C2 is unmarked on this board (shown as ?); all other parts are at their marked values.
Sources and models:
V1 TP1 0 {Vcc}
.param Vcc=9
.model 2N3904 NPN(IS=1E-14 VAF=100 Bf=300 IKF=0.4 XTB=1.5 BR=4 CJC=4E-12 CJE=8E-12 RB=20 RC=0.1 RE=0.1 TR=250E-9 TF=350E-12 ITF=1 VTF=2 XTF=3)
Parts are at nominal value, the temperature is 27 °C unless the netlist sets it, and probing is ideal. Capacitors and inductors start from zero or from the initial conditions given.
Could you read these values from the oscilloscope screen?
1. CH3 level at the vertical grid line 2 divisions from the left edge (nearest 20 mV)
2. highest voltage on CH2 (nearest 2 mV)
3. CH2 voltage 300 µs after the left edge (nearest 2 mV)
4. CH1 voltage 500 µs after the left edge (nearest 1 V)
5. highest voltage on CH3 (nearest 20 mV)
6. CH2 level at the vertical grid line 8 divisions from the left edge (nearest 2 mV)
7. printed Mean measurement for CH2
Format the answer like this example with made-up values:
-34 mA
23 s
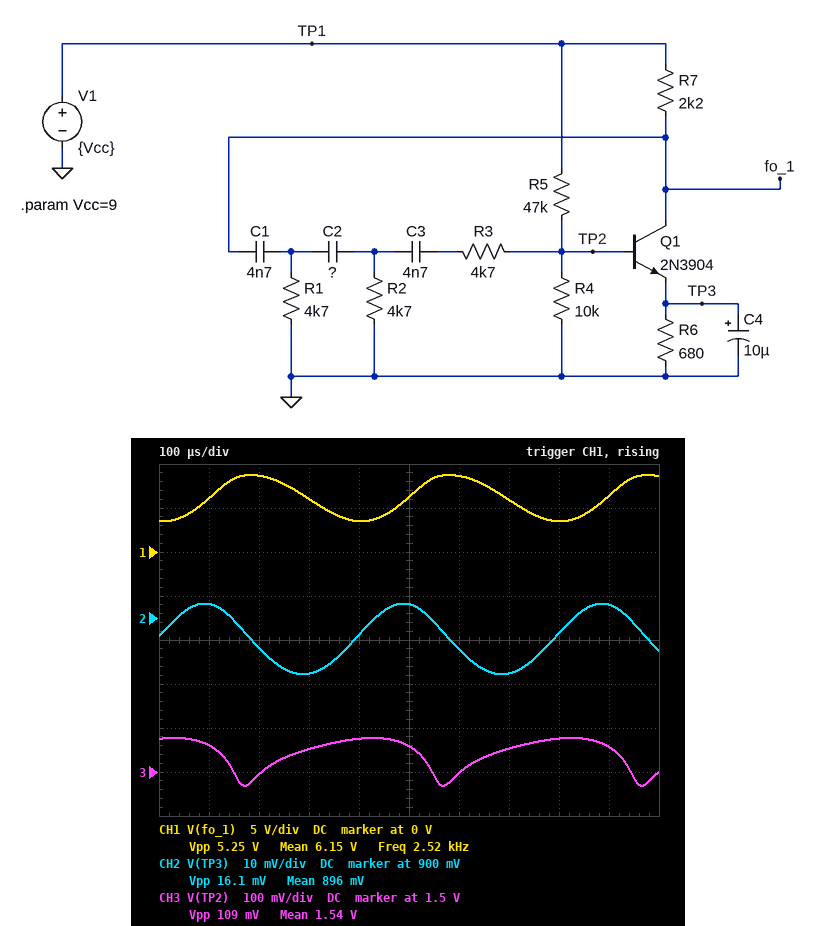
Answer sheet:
1.50 V
904 mV
888 mV
6 V
1.58 V
896 mV
896 mV
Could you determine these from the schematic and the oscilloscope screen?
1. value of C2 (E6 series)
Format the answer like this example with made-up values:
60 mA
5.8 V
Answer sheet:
3.3 nF
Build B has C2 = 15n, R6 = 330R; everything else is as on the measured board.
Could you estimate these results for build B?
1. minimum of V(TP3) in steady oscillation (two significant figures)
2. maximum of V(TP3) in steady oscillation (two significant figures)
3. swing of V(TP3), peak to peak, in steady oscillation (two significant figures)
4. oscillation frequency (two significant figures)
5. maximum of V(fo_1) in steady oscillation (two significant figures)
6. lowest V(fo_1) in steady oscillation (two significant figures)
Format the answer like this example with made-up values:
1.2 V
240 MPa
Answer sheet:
810 mV
830 mV
25 mV
1.6 kHz
6.3 V
910 mV
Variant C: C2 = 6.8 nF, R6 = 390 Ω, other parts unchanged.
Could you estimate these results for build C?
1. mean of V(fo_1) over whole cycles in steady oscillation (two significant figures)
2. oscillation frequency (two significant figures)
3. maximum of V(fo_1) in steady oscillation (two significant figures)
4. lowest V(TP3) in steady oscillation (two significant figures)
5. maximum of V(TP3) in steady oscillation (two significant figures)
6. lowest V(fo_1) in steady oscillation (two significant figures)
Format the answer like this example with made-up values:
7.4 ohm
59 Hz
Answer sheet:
4.3 V
2.1 kHz
8.0 V
820 mV
840 mV
910 mV
